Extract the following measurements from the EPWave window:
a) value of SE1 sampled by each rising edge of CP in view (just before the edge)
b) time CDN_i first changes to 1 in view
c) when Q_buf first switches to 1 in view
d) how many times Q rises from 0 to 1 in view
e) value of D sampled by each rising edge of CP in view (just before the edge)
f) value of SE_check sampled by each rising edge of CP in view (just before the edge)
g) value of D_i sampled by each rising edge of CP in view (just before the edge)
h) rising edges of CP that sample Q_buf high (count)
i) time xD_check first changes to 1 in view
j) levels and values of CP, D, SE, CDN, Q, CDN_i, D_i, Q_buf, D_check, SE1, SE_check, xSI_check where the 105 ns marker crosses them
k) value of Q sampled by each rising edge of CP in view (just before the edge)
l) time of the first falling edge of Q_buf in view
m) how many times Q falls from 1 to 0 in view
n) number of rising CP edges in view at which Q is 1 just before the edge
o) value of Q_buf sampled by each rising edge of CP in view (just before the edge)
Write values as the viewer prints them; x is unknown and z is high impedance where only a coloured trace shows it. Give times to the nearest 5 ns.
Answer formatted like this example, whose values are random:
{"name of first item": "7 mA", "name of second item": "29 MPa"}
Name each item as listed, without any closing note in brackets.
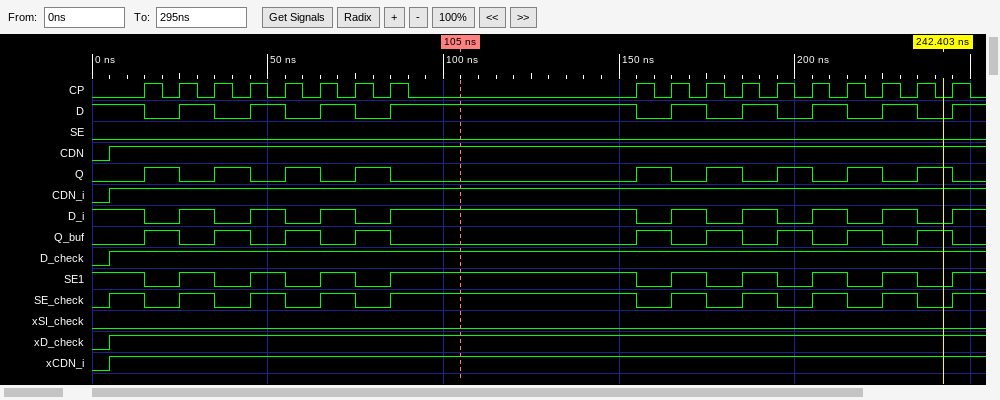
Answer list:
{"value of SE1 sampled by each rising edge of CP in view": "1 0 1 0 1 0 1 0 1 0 1 0 1 0 1 0 1 0", "time CDN_i first changes to 1 in view": "5 ns", "when Q_buf first switches to 1 in view": "15 ns", "how many times Q rises from 0 to 1 in view": "9", "value of D sampled by each rising edge of CP in view": "1 0 1 0 1 0 1 0 1 0 1 0 1 0 1 0 1 0", "value of SE_check sampled by each rising edge of CP in view": "1 0 1 0 1 0 1 0 1 0 1 0 1 0 1 0 1 0", "value of D_i sampled by each rising edge of CP in view": "1 0 1 0 1 0 1 0 1 0 1 0 1 0 1 0 1 0", "rising edges of CP that sample Q_buf high": "9", "time xD_check first changes to 1 in view": "5 ns", "levels and values of CP, D, SE, CDN, Q, CDN_i, D_i, Q_buf, D_check, SE1, SE_check, xSI_check where the 105 ns marker crosses them": "CP=0, D=1, SE=0, CDN=1, Q=0, CDN_i=1, D_i=1, Q_buf=0, D_check=1, SE1=1, SE_check=1, xSI_check=0", "value of Q sampled by each rising edge of CP in view": "0 1 0 1 0 1 0 1 0 1 0 1 0 1 0 1 0 1", "time of the first falling edge of Q_buf in view": "25 ns", "how many times Q falls from 1 to 0 in view": "9", "number of rising CP edges in view at which Q is 1 just before the edge": "9", "value of Q_buf sampled by each rising edge of CP in view": "0 1 0 1 0 1 0 1 0 1 0 1 0 1 0 1 0 1"}
